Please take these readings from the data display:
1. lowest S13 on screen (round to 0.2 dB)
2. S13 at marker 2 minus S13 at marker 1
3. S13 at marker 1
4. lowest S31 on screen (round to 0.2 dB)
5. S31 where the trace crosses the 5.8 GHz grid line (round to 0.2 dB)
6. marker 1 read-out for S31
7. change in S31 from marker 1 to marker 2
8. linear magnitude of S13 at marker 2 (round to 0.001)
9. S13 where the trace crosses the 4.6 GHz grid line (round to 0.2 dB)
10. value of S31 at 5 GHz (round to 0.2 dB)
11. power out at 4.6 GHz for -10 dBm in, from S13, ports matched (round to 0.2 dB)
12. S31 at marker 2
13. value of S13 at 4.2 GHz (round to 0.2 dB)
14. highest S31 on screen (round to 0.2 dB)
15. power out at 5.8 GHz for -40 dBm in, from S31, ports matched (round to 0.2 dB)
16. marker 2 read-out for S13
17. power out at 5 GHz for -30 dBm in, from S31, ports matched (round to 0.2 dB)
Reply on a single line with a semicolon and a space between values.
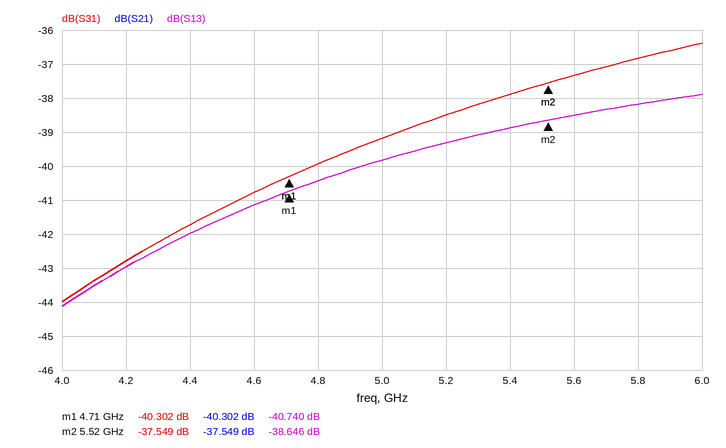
-44.2 dB; 2.094 dB; -40.740 dB; -44.0 dB; -36.8 dB; -40.302 dB; 2.753 dB; 0.012; -41.2 dB; -39.2 dB; -51.2 dBm; -37.549 dB; -43.0 dB; -36.4 dB; -76.8 dBm; -38.646 dB; -69.2 dBm
